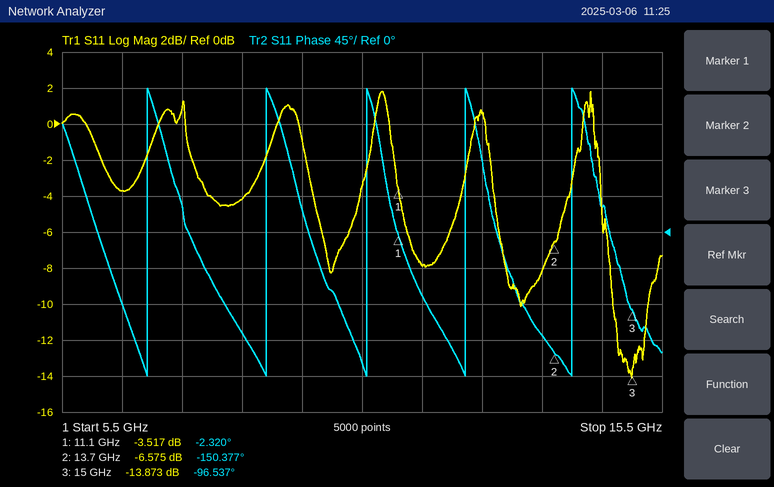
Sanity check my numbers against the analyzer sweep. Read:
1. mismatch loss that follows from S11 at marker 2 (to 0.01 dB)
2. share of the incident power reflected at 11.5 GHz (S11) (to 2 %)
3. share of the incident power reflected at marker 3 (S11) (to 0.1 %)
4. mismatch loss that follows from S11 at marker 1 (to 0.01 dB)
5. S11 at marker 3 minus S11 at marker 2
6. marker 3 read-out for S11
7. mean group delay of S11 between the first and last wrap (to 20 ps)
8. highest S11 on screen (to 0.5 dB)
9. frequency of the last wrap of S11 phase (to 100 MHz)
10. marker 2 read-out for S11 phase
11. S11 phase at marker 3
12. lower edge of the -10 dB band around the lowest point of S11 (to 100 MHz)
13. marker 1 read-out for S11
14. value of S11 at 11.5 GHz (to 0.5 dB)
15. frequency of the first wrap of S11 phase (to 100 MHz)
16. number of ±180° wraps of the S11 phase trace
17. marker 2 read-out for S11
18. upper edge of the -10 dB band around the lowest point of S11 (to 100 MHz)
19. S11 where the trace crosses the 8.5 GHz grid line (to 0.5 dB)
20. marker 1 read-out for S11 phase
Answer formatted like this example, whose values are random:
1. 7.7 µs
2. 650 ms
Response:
1. 1.08 dB
2. 16 %
3. 4.1 %
4. 2.56 dB
5. -7.298 dB
6. -13.873 dB
7. 560 ps
8. 2.0 dB
9. 14.0 GHz
10. -150.377°
11. -96.537°
12. 14.7 GHz
13. -3.517 dB
14. -8.0 dB
15. 6.9 GHz
16. 5
17. -6.575 dB
18. 15.3 GHz
19. -4.0 dB
20. -2.320°
